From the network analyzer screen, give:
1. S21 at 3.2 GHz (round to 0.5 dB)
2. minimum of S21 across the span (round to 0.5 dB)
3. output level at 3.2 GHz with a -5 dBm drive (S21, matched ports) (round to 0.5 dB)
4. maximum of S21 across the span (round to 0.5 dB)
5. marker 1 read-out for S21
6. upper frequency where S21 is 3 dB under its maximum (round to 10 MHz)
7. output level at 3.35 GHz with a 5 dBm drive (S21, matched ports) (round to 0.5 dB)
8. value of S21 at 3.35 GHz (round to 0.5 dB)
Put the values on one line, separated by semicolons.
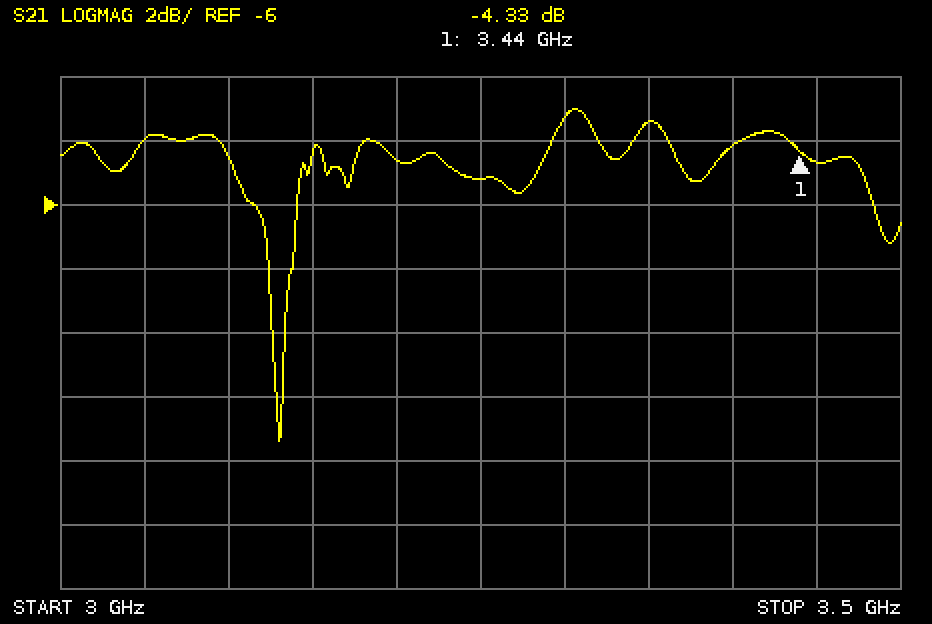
-4.5 dB; -13.5 dB; -9.5 dBm; -3.0 dB; -4.33 dB; 3.48 GHz; 1.5 dBm; -3.5 dB
